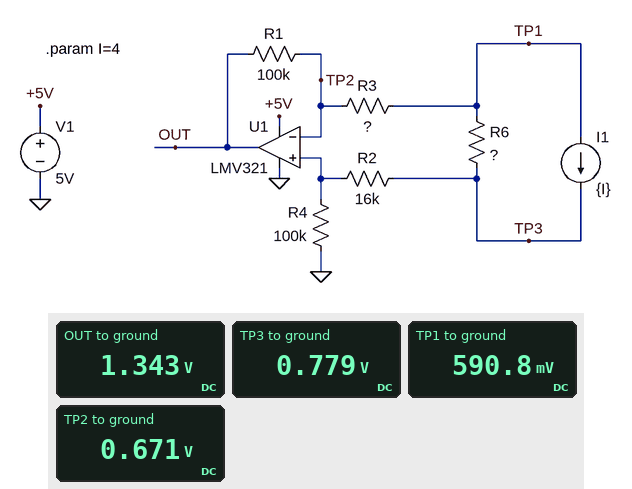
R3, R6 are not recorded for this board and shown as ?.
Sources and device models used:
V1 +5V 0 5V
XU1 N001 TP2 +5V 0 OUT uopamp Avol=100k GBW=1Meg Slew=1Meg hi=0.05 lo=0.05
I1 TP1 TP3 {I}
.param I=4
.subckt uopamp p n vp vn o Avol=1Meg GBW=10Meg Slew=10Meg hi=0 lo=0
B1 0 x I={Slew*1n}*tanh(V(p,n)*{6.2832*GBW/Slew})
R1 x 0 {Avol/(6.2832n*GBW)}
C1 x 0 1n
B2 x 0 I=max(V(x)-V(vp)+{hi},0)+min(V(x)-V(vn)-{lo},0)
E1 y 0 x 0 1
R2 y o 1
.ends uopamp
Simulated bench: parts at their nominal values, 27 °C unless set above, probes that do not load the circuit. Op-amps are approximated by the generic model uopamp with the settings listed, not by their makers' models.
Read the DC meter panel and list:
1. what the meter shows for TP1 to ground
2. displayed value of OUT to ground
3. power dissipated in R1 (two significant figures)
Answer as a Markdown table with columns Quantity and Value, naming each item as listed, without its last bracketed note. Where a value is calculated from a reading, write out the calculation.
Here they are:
| Quantity | Value |
|---|---|
| what the meter shows for TP1 to ground | 590.8 mV |
| displayed value of OUT to ground | 1.343 V |
| power dissipated in R1 | (1.343 V - 671 mV)^2 / 100 kΩ = 4.5 µW |
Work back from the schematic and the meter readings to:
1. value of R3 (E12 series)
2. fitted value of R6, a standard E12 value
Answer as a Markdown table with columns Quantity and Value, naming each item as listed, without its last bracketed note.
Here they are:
| Quantity | Value |
|---|---|
| value of R3 | 12 kΩ |
| fitted value of R6, a standard E12 value | 0.047 Ω |
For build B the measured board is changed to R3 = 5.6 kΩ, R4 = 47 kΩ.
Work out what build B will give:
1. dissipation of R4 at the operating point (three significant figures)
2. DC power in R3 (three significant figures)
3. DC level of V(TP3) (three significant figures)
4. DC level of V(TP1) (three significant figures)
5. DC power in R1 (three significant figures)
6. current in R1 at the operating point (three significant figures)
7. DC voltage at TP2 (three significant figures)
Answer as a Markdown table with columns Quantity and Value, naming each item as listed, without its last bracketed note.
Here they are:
| Quantity | Value |
|---|---|
| dissipation of R4 at the operating point | 3.56 µW |
| DC power in R3 | 424 nW |
| DC level of V(TP3) | 548 mV |
| DC level of V(TP1) | 360 mV |
| DC power in R1 | 7.57 µW |
| current in R1 at the operating point | 8.70 µA |
| DC voltage at TP2 | 409 mV |
